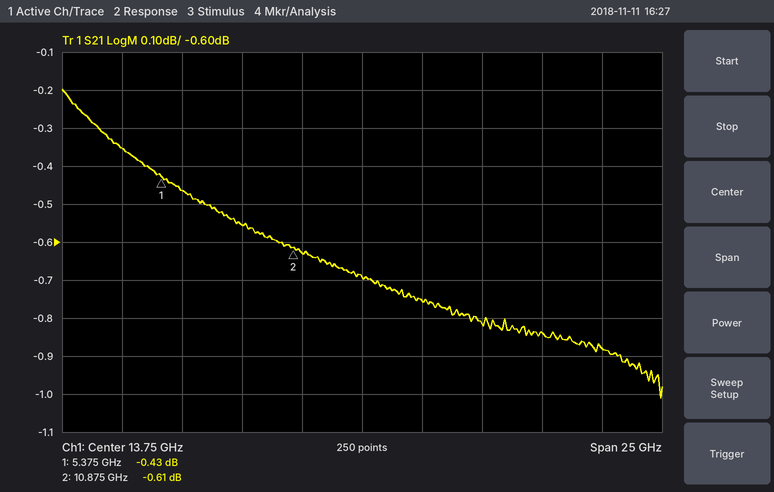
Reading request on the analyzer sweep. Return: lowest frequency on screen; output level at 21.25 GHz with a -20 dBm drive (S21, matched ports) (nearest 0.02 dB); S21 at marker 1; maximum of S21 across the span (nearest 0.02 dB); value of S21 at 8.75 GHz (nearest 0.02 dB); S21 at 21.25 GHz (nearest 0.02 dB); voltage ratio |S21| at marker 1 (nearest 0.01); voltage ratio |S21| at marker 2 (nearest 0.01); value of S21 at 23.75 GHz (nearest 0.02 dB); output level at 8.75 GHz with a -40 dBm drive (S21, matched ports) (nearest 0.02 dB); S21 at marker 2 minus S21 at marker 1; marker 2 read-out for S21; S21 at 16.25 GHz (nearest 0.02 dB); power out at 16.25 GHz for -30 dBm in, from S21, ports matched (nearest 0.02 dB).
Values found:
1.25 GHz
-20.84 dBm
-0.43 dB
-0.20 dB
-0.56 dB
-0.84 dB
0.95
0.93
-0.88 dB
-40.56 dBm
-0.18 dB
-0.61 dB
-0.76 dB
-30.76 dBm
